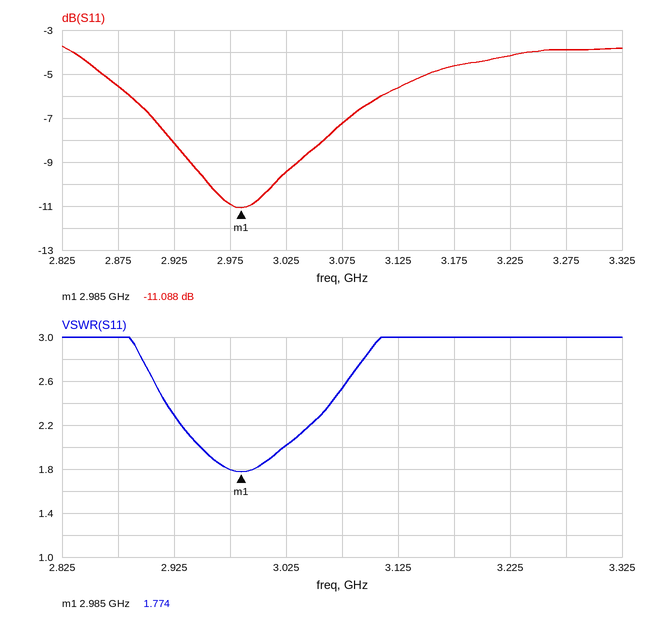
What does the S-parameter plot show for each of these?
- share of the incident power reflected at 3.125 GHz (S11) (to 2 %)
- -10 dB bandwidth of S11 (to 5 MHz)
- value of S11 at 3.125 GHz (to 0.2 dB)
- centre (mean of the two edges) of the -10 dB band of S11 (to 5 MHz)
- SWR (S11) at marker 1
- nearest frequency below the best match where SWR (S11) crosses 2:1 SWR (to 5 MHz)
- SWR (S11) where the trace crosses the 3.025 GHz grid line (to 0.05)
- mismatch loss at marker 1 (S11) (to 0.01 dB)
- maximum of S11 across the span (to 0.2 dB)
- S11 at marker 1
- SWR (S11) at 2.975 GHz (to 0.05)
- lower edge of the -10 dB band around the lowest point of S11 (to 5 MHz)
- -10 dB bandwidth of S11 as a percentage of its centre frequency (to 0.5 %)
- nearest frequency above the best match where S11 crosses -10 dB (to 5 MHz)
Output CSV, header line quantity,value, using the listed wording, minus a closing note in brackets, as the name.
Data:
quantity,value
share of the incident power reflected at 3.125 GHz (S11),28 %
-10 dB bandwidth of S11,60 MHz
value of S11 at 3.125 GHz,-5.6 dB
centre (mean of the two edges) of the -10 dB band of S11,2.985 GHz
SWR (S11) at marker 1,1.774
nearest frequency below the best match where SWR (S11) crosses 2:1 SWR,2.950 GHz
SWR (S11) where the trace crosses the 3.025 GHz grid line,2.00
mismatch loss at marker 1 (S11),0.35 dB
maximum of S11 across the span,-3.8 dB
S11 at marker 1,-11.088 dB
SWR (S11) at 2.975 GHz,1.80
lower edge of the -10 dB band around the lowest point of S11,2.955 GHz
-10 dB bandwidth of S11 as a percentage of its centre frequency,2.0 %
nearest frequency above the best match where S11 crosses -10 dB,3.015 GHz
